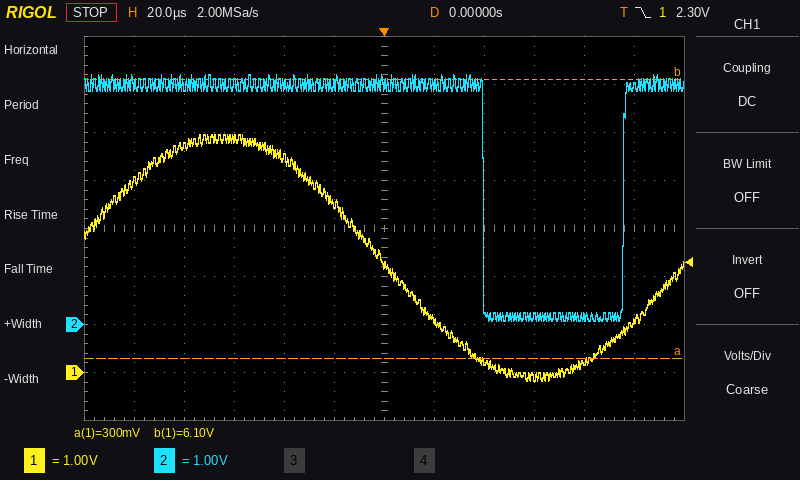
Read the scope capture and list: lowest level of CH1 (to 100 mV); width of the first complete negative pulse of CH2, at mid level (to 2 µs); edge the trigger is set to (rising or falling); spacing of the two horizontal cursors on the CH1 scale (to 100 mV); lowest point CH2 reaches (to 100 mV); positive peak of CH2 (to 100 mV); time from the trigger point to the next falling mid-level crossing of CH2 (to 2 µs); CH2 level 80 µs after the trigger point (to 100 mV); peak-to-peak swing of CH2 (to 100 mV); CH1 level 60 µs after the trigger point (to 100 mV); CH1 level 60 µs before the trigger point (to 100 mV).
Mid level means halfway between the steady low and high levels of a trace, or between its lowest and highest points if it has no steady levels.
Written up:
-200 mV
56 µs
falling
5.8 V
100 mV
5.2 V
40 µs
200 mV
5.1 V
-100 mV
4.9 V
